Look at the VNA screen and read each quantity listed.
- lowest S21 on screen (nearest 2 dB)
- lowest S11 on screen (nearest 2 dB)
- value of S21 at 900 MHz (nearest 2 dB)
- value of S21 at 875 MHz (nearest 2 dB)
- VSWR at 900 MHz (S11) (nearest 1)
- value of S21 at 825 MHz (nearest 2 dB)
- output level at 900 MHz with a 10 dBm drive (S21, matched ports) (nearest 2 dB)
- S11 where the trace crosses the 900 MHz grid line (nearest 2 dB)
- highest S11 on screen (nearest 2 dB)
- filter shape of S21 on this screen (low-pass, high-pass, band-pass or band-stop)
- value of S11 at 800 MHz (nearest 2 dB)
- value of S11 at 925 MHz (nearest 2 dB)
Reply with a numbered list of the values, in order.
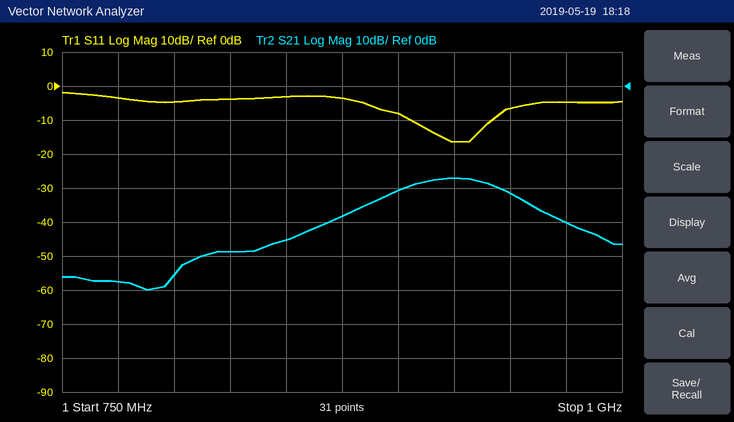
1. -60 dB
2. -16 dB
3. -30 dB
4. -38 dB
5. 2
6. -48 dB
7. -20 dBm
8. -8 dB
9. -2 dB
10. band-pass
11. -4 dB
12. -16 dB
